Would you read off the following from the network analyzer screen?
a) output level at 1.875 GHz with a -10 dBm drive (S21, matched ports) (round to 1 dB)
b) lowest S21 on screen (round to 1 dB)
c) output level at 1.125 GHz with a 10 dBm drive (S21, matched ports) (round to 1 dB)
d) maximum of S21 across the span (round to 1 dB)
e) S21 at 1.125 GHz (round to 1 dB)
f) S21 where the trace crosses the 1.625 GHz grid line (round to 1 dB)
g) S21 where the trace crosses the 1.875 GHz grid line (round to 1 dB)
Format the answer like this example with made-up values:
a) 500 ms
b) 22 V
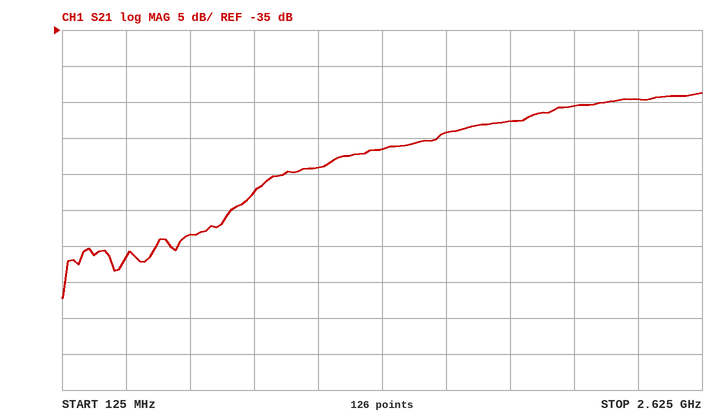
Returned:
a) -58 dBm
b) -72 dB
c) -44 dBm
d) -44 dB
e) -54 dB
f) -49 dB
g) -48 dB
